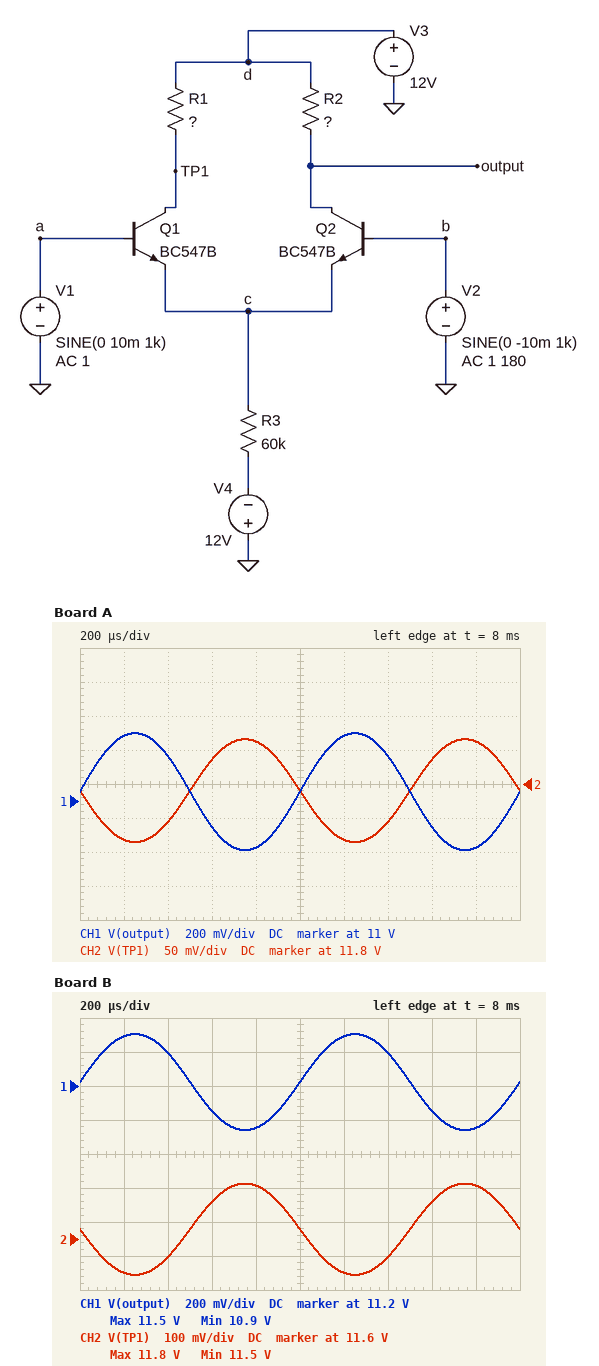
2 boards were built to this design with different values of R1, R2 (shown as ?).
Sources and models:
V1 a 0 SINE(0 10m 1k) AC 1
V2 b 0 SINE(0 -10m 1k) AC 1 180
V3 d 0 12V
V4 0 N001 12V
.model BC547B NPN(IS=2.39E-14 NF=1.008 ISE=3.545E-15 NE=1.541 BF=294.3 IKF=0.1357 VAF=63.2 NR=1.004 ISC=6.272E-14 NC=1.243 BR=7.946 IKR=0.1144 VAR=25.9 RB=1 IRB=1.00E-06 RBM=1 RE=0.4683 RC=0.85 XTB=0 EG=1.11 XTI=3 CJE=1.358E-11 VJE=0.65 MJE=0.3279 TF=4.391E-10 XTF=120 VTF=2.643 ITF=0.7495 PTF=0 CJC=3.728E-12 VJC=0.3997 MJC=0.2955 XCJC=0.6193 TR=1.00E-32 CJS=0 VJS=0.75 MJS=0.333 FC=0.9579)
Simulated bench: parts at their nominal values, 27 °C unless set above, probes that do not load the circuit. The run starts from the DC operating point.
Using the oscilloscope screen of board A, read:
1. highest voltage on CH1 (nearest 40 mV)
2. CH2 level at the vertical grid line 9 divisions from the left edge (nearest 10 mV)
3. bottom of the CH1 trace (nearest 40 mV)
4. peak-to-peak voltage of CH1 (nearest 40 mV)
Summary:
11.40 V
11.86 V
10.72 V
680 mV
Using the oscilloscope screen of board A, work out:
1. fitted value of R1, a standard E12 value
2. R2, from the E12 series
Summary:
2.2 kΩ
10 kΩ
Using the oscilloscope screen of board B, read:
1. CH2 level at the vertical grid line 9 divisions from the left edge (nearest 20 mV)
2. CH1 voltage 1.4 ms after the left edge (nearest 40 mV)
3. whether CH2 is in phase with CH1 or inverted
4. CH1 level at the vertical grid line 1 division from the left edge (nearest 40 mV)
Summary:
11.76 V
11.40 V
inverted
11.48 V
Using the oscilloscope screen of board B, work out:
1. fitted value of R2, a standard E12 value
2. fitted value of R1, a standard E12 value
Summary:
8.2 kΩ
3.9 kΩ
